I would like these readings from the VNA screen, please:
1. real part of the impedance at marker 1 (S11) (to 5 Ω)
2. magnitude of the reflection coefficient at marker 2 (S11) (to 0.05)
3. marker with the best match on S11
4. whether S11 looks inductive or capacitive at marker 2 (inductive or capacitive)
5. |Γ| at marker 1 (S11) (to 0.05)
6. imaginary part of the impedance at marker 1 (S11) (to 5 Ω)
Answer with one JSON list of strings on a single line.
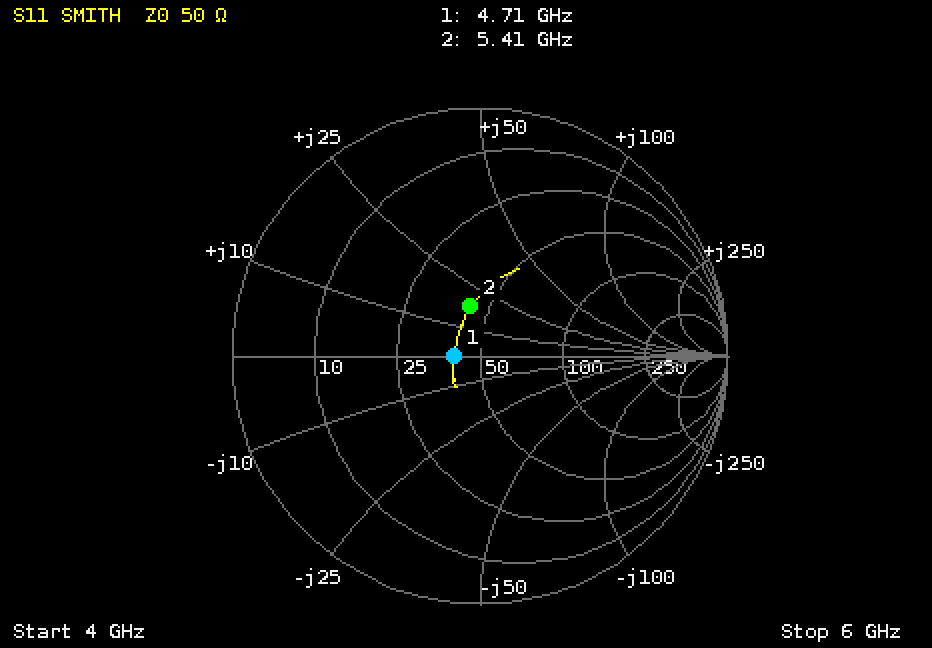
["40 Ω", "0.20", "marker 1", "inductive", "0.10", "0 Ω"]
